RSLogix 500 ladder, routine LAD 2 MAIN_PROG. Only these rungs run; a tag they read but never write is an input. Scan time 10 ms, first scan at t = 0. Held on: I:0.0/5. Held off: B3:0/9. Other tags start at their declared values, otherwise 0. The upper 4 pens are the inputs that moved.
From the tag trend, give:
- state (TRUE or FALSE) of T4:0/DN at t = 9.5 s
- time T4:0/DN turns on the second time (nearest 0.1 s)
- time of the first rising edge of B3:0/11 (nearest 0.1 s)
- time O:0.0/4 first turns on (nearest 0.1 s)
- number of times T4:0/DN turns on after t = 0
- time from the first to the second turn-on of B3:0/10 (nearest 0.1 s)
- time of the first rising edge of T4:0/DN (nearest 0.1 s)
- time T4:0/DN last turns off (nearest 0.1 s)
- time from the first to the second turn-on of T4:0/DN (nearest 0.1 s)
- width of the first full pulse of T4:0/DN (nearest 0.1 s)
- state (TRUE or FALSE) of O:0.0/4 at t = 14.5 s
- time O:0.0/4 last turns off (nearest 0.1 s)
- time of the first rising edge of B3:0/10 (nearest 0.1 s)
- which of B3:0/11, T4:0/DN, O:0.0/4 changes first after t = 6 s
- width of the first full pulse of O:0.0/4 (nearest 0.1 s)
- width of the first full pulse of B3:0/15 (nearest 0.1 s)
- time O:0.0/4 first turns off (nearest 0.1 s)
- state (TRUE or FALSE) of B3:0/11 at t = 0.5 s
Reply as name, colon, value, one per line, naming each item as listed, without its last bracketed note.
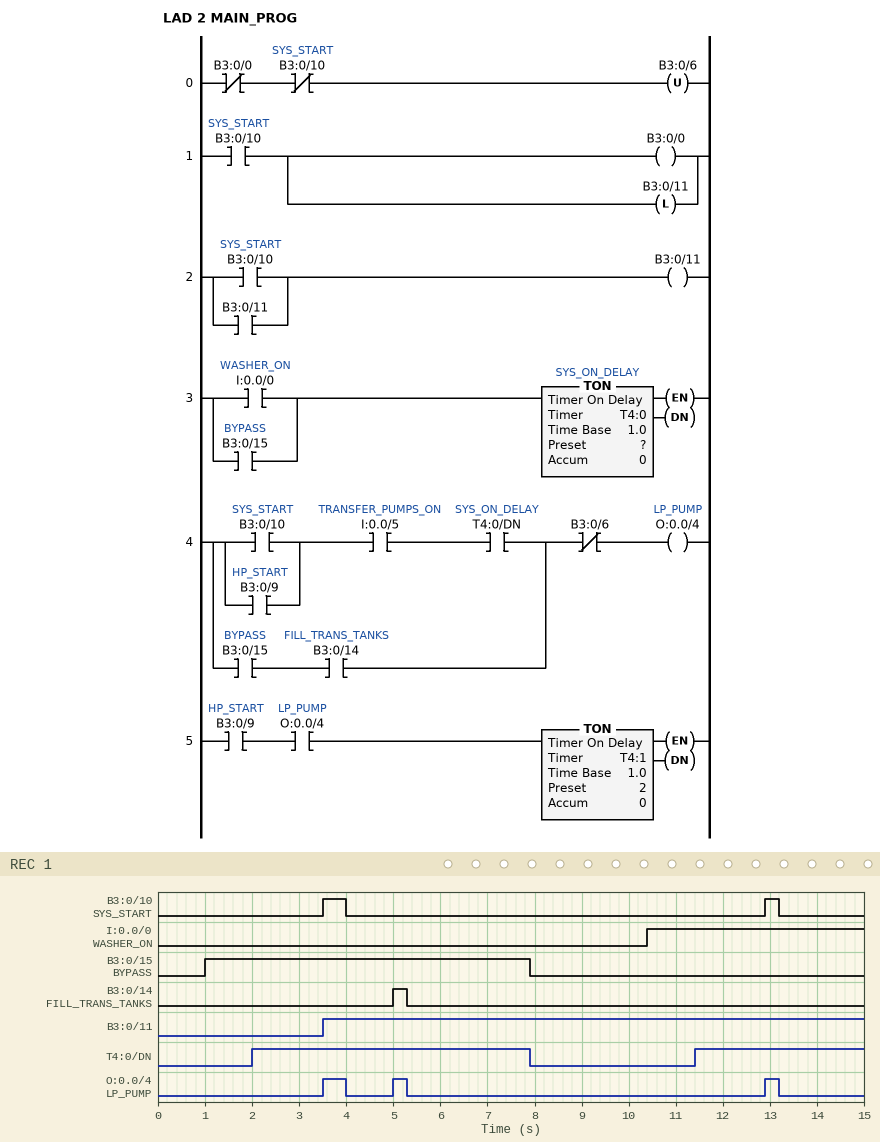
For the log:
state (TRUE or FALSE) of T4:0/DN at t = 9.5 s: FALSE
time T4:0/DN turns on the second time: 11.4 s
time of the first rising edge of B3:0/11: 3.5 s
time O:0.0/4 first turns on: 3.5 s
number of times T4:0/DN turns on after t = 0: 2
time from the first to the second turn-on of B3:0/10: 9.4 s
time of the first rising edge of T4:0/DN: 2.0 s
time T4:0/DN last turns off: 7.9 s
time from the first to the second turn-on of T4:0/DN: 9.4 s
width of the first full pulse of T4:0/DN: 5.9 s
state (TRUE or FALSE) of O:0.0/4 at t = 14.5 s: FALSE
time O:0.0/4 last turns off: 13.2 s
time of the first rising edge of B3:0/10: 3.5 s
which of B3:0/11, T4:0/DN, O:0.0/4 changes first after t = 6 s: T4:0/DN
width of the first full pulse of O:0.0/4: 0.5 s
width of the first full pulse of B3:0/15: 6.9 s
time O:0.0/4 first turns off: 4.0 s
state (TRUE or FALSE) of B3:0/11 at t = 0.5 s: FALSE
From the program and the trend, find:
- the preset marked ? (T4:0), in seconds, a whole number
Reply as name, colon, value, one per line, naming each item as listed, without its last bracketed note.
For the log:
the preset marked ? (T4:0), in seconds, a whole number: 1 s
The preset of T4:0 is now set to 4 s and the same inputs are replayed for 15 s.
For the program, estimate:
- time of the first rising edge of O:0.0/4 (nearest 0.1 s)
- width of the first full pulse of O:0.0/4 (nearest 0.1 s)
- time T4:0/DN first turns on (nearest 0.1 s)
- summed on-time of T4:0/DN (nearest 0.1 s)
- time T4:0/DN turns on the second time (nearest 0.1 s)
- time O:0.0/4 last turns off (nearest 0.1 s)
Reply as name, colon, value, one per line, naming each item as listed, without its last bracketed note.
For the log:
time of the first rising edge of O:0.0/4: 5.0 s
width of the first full pulse of O:0.0/4: 0.3 s
time T4:0/DN first turns on: 5.0 s
summed on-time of T4:0/DN: 3.5 s
time T4:0/DN turns on the second time: 14.4 s
time O:0.0/4 last turns off: 5.3 s
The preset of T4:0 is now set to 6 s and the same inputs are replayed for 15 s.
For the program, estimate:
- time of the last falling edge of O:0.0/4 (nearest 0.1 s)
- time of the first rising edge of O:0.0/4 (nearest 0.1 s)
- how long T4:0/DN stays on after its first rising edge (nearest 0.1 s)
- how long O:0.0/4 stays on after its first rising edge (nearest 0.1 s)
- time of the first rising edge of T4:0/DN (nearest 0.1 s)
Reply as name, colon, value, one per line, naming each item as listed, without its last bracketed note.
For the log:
time of the last falling edge of O:0.0/4: 5.3 s
time of the first rising edge of O:0.0/4: 5.0 s
how long T4:0/DN stays on after its first rising edge: 0.9 s
how long O:0.0/4 stays on after its first rising edge: 0.3 s
time of the first rising edge of T4:0/DN: 7.0 s
